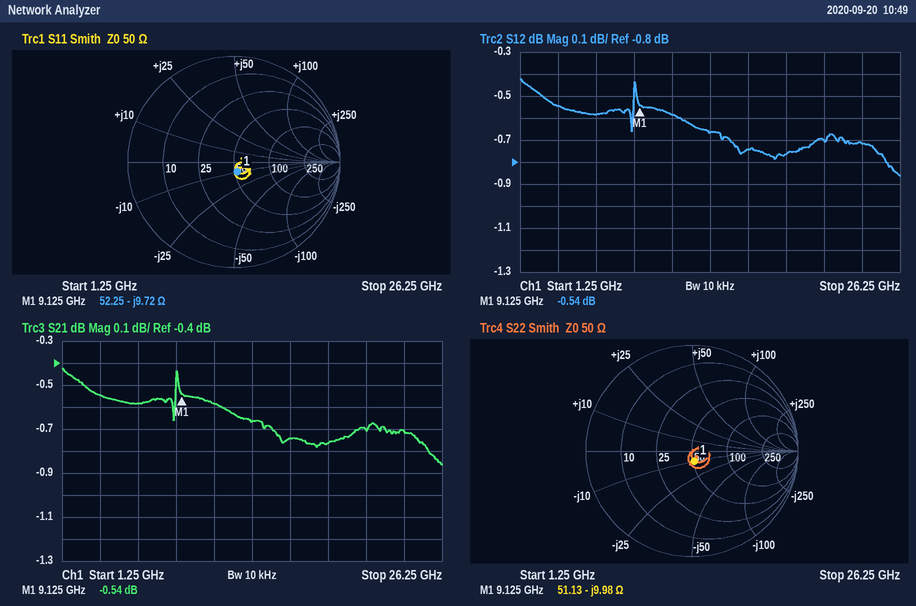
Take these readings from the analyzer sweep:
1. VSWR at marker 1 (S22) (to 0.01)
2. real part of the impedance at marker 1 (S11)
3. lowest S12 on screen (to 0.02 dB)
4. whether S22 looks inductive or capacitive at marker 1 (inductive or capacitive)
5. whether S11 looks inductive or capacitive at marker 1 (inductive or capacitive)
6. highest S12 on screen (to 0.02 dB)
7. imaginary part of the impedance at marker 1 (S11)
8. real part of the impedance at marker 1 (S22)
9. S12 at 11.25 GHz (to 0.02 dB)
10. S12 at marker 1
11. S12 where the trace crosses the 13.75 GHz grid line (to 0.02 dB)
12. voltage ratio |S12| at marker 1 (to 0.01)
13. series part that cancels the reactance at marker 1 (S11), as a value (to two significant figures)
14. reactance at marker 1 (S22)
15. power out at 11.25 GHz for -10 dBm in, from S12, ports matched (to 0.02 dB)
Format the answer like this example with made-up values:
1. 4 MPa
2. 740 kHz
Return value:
1. 1.22
2. 52.25 Ω
3. -0.86 dB
4. capacitive
5. capacitive
6. -0.42 dB
7. -9.72 Ω
8. 51.13 Ω
9. -0.58 dB
10. -0.54 dB
11. -0.66 dB
12. 0.94
13. 170 pH
14. -9.98 Ω
15. -10.58 dBm
